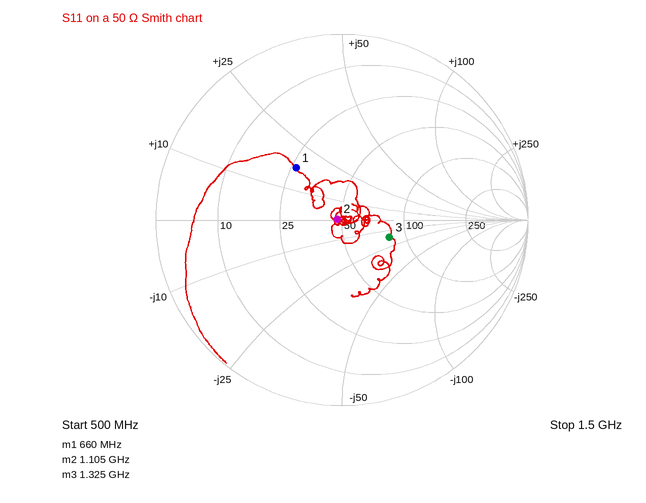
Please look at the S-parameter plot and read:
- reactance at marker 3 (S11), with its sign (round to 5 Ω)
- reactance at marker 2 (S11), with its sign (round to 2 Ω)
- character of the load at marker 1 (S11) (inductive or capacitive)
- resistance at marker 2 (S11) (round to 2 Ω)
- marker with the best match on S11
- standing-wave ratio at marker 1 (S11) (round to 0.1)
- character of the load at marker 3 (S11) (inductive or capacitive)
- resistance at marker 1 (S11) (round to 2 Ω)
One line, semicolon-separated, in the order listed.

-15 Ω; 0 Ω; inductive; 48 Ω; marker 2; 2.2; capacitive; 26 Ω
